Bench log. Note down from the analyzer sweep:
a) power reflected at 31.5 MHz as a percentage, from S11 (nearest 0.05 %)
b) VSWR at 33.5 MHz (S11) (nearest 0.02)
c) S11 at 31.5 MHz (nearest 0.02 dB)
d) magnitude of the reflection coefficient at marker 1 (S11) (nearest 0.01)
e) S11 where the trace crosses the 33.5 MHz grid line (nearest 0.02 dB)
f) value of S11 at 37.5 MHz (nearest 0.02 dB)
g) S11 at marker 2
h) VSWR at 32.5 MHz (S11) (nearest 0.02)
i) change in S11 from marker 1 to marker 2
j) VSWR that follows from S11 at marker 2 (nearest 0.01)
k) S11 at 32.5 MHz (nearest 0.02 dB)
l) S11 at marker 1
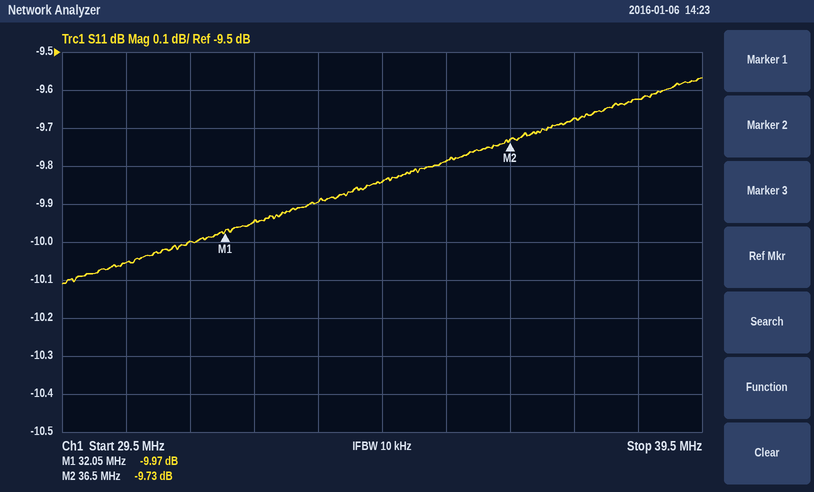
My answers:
10.00 %
1.94
-10.00 dB
0.32
-9.90 dB
-9.68 dB
-9.73 dB
1.94
0.24 dB
1.97
-9.94 dB
-9.97 dB
